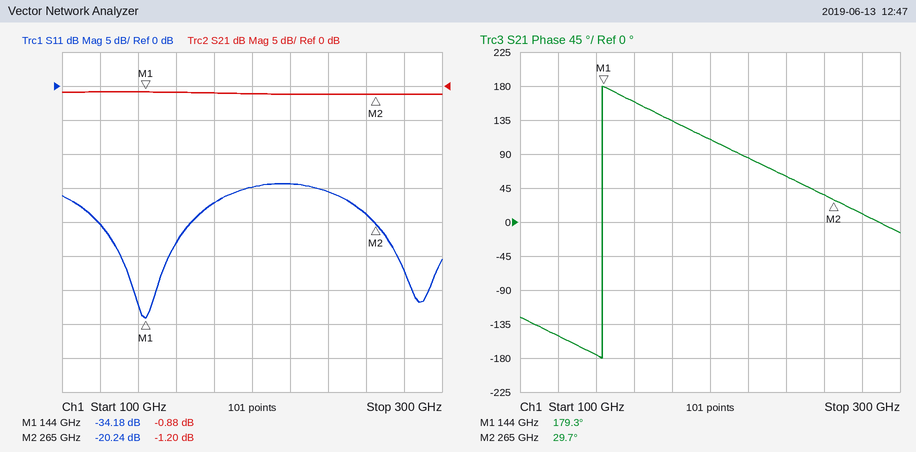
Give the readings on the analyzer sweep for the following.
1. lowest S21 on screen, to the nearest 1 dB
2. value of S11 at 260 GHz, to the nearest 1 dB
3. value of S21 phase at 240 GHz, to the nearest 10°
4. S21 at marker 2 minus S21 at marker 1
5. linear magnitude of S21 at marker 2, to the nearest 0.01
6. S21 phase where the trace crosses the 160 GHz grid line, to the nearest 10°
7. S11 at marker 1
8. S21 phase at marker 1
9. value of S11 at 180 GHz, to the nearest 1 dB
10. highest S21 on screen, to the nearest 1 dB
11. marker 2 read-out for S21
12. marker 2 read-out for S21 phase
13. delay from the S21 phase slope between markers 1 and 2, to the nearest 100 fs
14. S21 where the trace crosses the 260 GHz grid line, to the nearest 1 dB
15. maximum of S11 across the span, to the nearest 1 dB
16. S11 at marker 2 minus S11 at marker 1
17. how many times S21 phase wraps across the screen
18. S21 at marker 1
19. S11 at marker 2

-1 dB
-19 dB
60°
-0.32 dB
0.87
160°
-34.18 dB
179.3°
-17 dB
-1 dB
-1.20 dB
29.7°
3.4 ps
-1 dB
-14 dB
13.94 dB
1
-0.88 dB
-20.24 dB
